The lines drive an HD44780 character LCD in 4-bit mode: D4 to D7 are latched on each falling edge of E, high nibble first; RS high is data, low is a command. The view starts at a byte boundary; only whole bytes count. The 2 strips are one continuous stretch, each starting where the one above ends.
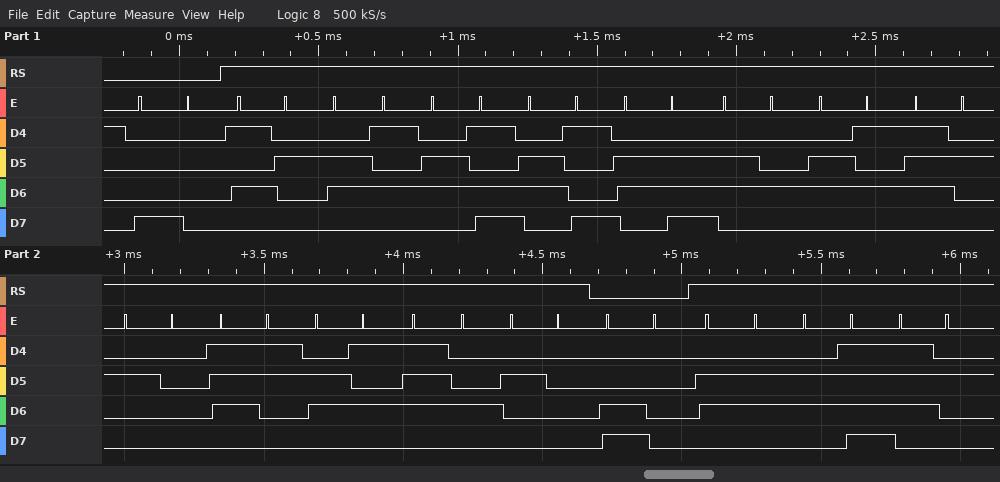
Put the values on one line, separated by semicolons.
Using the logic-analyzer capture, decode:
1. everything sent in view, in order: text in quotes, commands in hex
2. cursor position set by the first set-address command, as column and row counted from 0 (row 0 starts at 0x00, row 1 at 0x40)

0x80 "Reminder set " 0xC0 "for"; column 0, row 0
